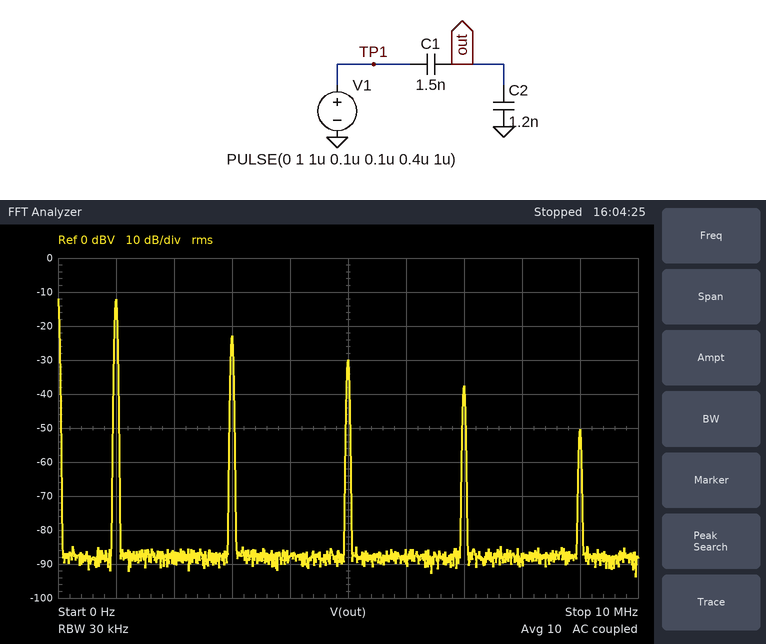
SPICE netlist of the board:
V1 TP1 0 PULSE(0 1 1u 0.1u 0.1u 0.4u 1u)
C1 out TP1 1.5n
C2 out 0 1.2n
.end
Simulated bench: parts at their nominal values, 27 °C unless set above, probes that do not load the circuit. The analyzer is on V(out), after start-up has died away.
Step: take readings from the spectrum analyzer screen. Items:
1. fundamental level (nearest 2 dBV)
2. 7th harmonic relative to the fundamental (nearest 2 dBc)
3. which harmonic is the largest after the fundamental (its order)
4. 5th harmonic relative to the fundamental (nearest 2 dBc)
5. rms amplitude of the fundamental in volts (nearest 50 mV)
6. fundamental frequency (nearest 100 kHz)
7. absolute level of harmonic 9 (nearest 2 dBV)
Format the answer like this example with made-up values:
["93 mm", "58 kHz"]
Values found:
["-12 dBV", "-26 dBc", "3", "-18 dBc", "250 mV", "1.0 MHz", "-50 dBV"]
